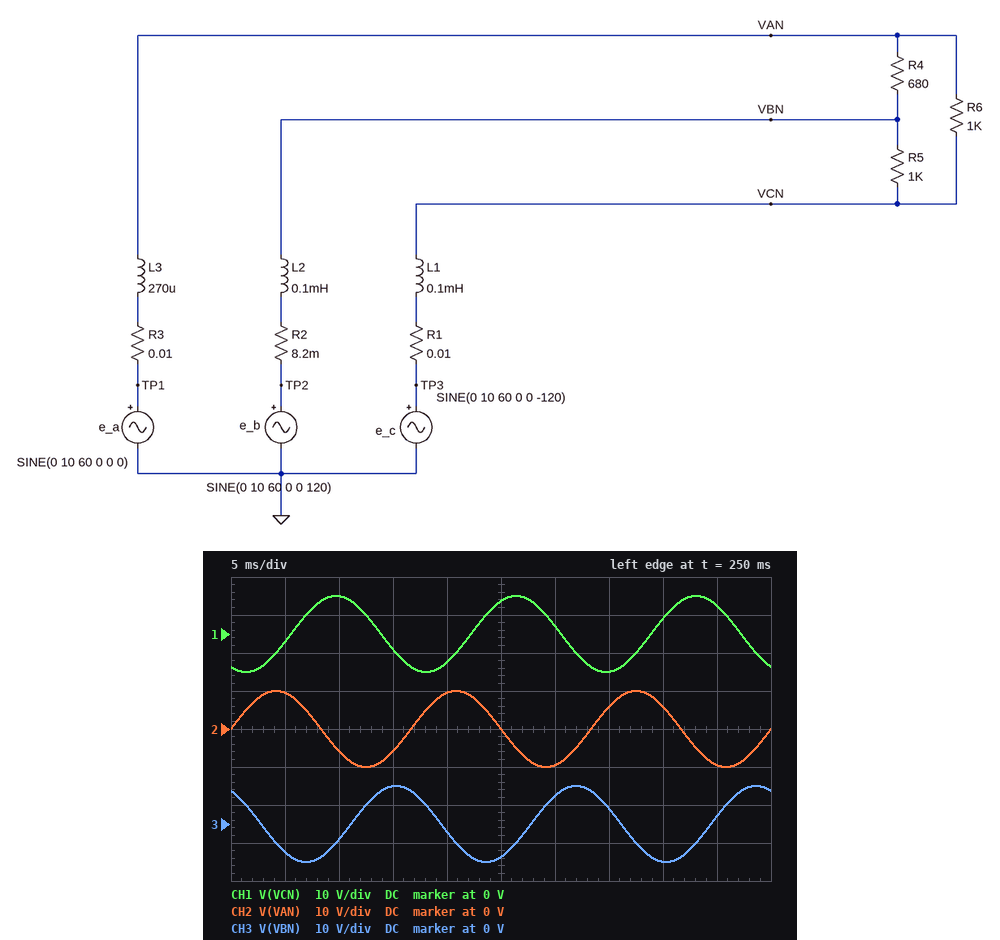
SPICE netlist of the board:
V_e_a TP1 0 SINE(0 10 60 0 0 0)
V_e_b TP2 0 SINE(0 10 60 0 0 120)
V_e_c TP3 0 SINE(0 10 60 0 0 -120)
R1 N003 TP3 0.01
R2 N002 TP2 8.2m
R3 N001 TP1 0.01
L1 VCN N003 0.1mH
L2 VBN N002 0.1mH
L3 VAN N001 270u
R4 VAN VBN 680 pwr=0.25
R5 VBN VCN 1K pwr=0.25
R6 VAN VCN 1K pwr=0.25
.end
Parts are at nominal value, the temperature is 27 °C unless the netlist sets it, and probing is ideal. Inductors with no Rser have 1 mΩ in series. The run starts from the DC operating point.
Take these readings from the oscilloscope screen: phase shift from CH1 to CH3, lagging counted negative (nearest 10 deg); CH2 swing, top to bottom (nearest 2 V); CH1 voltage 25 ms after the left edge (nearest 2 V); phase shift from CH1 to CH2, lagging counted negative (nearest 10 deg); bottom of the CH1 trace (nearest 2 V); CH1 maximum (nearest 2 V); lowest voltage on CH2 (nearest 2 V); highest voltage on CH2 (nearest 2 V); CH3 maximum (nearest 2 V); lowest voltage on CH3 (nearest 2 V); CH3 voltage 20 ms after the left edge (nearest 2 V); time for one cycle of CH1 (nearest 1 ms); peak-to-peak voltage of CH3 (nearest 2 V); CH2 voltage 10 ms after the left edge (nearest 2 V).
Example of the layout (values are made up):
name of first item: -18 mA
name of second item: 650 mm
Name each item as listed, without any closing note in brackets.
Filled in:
phase shift from CH1 to CH3, lagging counted negative: -120 deg
CH2 swing, top to bottom: 20 V
CH1 voltage 25 ms after the left edge: 8 V
phase shift from CH1 to CH2, lagging counted negative: 120 deg
bottom of the CH1 trace: -10 V
CH1 maximum: 10 V
lowest voltage on CH2: -10 V
highest voltage on CH2: 10 V
CH3 maximum: 10 V
lowest voltage on CH3: -10 V
CH3 voltage 20 ms after the left edge: -2 V
time for one cycle of CH1: 17 ms
peak-to-peak voltage of CH3: 20 V
CH2 voltage 10 ms after the left edge: -6 V
